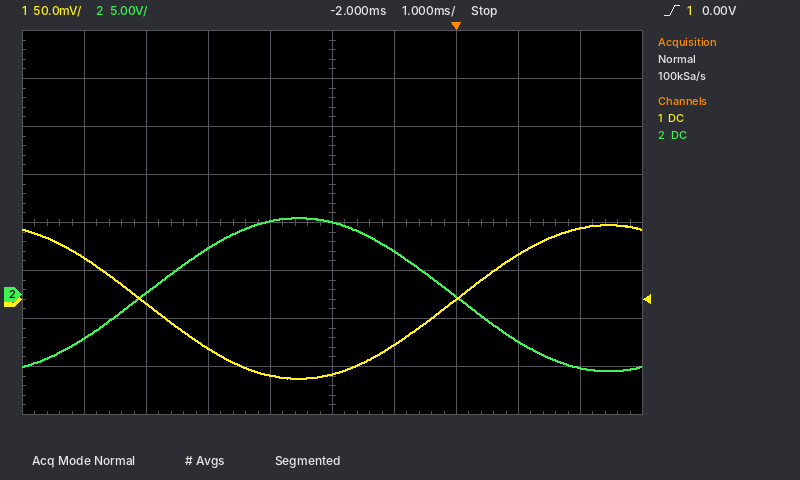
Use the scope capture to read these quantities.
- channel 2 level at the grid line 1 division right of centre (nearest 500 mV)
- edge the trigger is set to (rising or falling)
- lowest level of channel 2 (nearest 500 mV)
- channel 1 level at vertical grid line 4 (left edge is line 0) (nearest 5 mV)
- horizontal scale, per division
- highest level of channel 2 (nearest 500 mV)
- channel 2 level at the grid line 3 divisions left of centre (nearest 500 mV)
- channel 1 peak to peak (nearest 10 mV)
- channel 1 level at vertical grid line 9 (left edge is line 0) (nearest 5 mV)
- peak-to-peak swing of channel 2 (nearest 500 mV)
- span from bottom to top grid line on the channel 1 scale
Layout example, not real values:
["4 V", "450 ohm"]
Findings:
["4.5 V", "rising", "-8.0 V", "-80 mV", "1 ms", "8.0 V", "0.0 V", "160 mV", "75 mV", "16.0 V", "400 mV"]
